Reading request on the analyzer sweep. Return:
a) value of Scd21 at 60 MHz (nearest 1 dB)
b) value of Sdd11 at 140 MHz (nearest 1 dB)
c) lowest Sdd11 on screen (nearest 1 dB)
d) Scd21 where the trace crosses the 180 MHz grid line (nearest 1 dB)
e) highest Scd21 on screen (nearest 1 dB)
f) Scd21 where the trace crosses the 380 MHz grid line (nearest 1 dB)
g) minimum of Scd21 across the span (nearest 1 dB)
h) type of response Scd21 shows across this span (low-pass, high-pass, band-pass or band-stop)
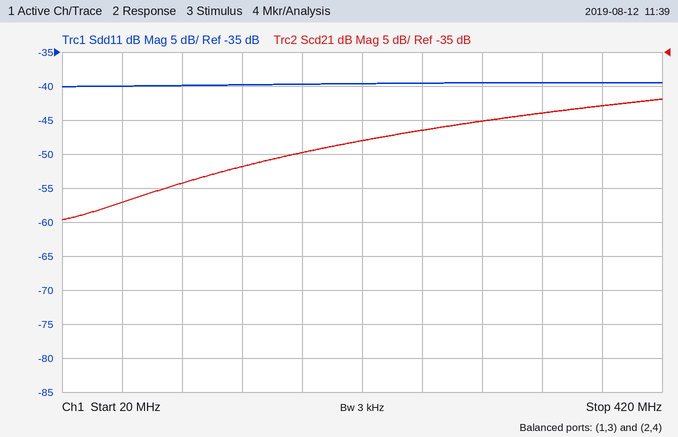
-57 dB
-40 dB
-40 dB
-50 dB
-42 dB
-43 dB
-60 dB
high-pass
